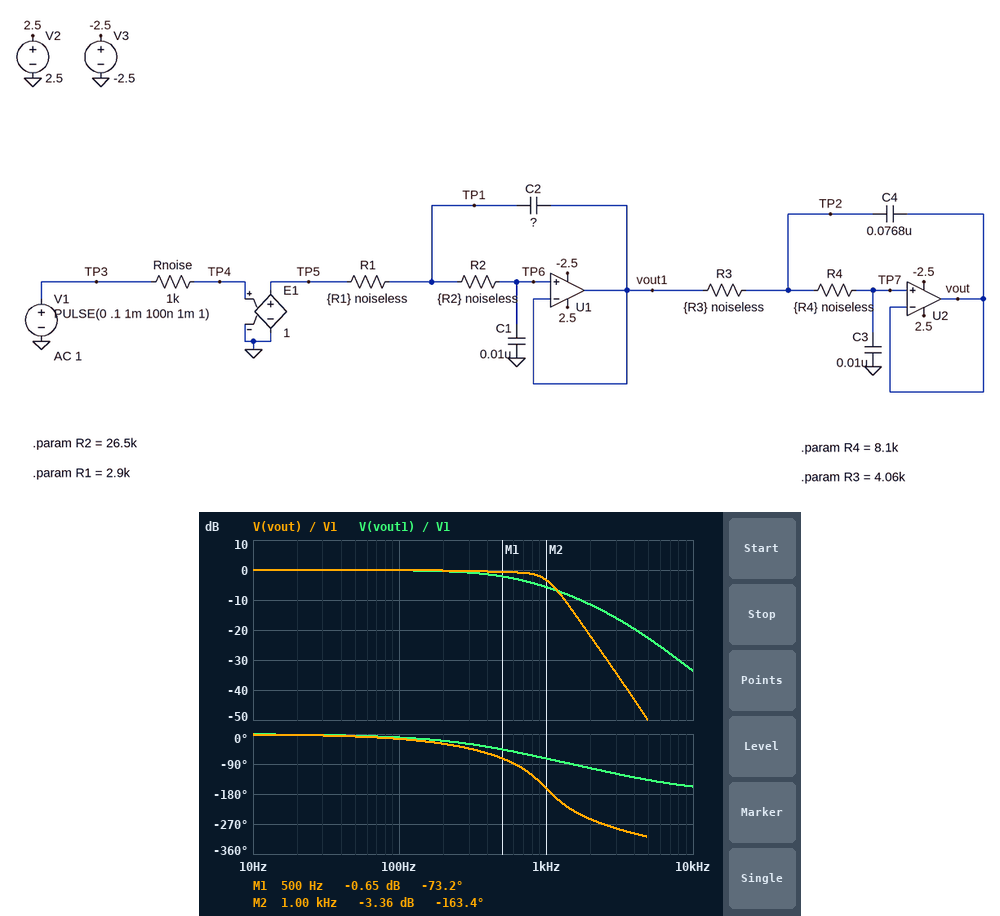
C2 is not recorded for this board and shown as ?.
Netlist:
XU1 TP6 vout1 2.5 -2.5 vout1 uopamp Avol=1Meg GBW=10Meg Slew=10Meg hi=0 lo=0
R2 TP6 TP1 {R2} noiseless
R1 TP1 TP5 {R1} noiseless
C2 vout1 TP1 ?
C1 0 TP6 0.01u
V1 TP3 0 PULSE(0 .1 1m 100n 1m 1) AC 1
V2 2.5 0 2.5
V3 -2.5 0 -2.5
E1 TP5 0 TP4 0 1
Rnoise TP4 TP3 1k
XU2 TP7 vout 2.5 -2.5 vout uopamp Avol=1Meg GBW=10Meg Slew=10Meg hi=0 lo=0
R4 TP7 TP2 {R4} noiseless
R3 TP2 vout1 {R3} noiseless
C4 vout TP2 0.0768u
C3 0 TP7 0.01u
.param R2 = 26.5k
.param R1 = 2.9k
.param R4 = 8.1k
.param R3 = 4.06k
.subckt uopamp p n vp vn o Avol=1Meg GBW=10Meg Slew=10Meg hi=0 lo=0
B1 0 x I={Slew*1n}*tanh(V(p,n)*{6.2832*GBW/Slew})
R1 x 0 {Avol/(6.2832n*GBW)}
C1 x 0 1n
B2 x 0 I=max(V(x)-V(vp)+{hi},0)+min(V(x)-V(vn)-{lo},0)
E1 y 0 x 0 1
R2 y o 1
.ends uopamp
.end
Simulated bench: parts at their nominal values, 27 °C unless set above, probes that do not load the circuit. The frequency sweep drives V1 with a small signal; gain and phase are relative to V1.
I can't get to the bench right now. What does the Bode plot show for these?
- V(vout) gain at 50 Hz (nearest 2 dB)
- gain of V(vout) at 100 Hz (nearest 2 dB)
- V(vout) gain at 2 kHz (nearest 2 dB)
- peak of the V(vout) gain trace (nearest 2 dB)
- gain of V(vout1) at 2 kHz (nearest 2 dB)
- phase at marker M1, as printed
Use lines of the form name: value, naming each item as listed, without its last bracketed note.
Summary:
V(vout) gain at 50 Hz: 0 dB
gain of V(vout) at 100 Hz: 0 dB
V(vout) gain at 2 kHz: -22 dB
peak of the V(vout) gain trace: 0 dB
gain of V(vout1) at 2 kHz: -12 dB
phase at marker M1, as printed: -73.2 deg
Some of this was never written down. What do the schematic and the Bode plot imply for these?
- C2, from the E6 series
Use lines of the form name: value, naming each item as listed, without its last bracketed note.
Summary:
C2, from the E6 series: 15 nF
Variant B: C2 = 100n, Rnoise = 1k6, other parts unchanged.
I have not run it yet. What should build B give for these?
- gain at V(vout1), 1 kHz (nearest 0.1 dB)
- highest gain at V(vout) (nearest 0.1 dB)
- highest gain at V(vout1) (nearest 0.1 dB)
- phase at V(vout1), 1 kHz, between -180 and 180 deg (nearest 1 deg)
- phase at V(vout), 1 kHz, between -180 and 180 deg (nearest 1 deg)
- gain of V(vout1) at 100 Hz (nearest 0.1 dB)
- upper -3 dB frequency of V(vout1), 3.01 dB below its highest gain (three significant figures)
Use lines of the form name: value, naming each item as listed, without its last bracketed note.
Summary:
gain at V(vout1), 1 kHz: -8.8 dB
highest gain at V(vout): 2.0 dB
highest gain at V(vout1): 0.9 dB
phase at V(vout1), 1 kHz, between -180 and 180 deg: -138 deg
phase at V(vout), 1 kHz, between -180 and 180 deg: 132 deg
gain of V(vout1) at 100 Hz: 0.1 dB
upper -3 dB frequency of V(vout1), 3.01 dB below its highest gain: 664 Hz
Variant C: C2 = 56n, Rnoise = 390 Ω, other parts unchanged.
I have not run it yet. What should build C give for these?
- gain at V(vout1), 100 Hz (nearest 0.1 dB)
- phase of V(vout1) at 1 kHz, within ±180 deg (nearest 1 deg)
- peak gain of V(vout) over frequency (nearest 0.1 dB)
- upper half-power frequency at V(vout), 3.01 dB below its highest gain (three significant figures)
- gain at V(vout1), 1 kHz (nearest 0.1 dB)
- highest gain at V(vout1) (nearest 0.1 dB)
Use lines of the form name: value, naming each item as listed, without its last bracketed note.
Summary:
gain at V(vout1), 100 Hz: 0 dB
phase of V(vout1) at 1 kHz, within ±180 deg: -111 deg
peak gain of V(vout) over frequency: 0.8 dB
upper half-power frequency at V(vout), 3.01 dB below its highest gain: 933 Hz
gain at V(vout1), 1 kHz: -5.9 dB
highest gain at V(vout1): 0 dB
